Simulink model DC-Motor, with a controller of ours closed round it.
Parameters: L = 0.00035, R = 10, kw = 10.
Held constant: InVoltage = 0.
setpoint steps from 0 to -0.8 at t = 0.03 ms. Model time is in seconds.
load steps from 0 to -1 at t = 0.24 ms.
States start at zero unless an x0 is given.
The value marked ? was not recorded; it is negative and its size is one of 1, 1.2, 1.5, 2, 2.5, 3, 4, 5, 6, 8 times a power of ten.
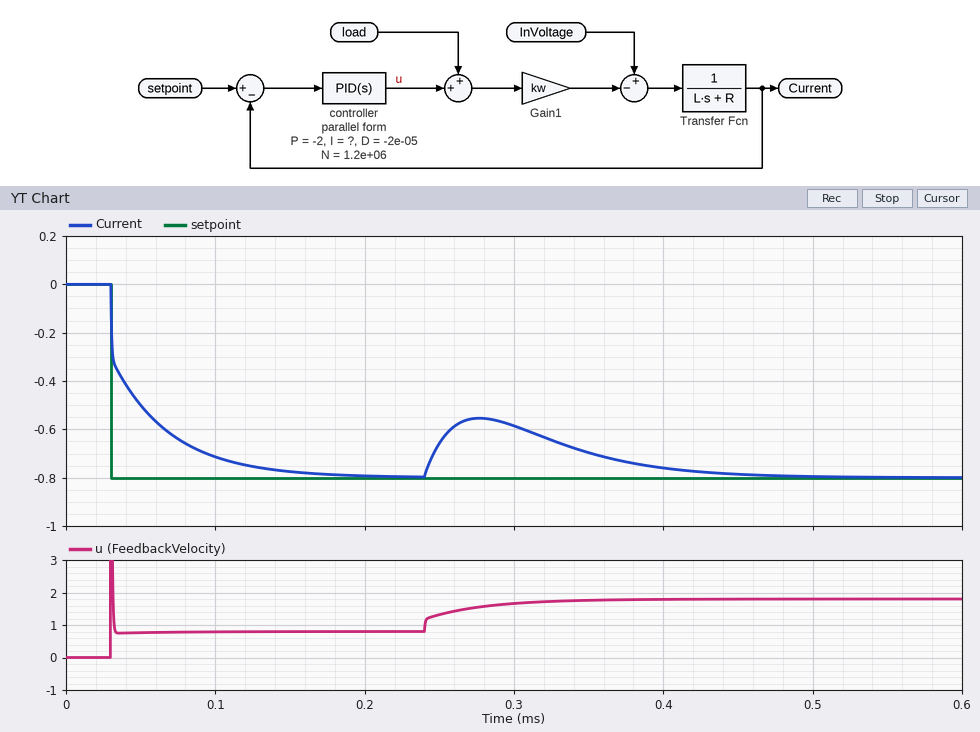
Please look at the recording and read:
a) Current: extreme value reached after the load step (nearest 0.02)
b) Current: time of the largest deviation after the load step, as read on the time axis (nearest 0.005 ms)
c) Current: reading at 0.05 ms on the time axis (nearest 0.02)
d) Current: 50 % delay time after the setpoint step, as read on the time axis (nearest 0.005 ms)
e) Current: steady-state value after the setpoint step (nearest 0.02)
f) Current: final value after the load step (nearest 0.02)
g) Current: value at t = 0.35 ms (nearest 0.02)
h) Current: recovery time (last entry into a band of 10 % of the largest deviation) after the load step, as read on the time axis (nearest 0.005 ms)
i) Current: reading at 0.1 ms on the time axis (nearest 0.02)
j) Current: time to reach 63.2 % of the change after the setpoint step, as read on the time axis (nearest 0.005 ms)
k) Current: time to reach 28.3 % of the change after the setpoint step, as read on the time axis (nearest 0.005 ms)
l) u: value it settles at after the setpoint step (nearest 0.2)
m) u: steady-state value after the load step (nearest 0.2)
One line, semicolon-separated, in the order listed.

-0.56; 0.275 ms; -0.50; 0.040 ms; -0.80; -0.80; -0.70; 0.425 ms; -0.72; 0.050 ms; 0.030 ms; 0.8; 1.8
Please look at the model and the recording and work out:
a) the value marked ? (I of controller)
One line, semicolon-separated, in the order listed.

-40000
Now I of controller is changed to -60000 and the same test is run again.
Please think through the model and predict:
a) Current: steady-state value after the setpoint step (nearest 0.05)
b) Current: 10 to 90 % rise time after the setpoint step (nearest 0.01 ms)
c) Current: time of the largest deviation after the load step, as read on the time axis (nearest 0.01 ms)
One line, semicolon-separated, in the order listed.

-0.80; 0.05 ms; 0.27 ms
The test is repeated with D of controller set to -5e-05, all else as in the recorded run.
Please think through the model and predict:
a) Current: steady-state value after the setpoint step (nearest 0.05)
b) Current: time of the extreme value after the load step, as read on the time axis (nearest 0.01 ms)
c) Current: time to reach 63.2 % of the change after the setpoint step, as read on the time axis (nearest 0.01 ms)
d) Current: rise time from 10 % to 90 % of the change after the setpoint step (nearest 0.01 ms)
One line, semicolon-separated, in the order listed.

-0.80; 0.29 ms; 0.04 ms; 0.09 ms
